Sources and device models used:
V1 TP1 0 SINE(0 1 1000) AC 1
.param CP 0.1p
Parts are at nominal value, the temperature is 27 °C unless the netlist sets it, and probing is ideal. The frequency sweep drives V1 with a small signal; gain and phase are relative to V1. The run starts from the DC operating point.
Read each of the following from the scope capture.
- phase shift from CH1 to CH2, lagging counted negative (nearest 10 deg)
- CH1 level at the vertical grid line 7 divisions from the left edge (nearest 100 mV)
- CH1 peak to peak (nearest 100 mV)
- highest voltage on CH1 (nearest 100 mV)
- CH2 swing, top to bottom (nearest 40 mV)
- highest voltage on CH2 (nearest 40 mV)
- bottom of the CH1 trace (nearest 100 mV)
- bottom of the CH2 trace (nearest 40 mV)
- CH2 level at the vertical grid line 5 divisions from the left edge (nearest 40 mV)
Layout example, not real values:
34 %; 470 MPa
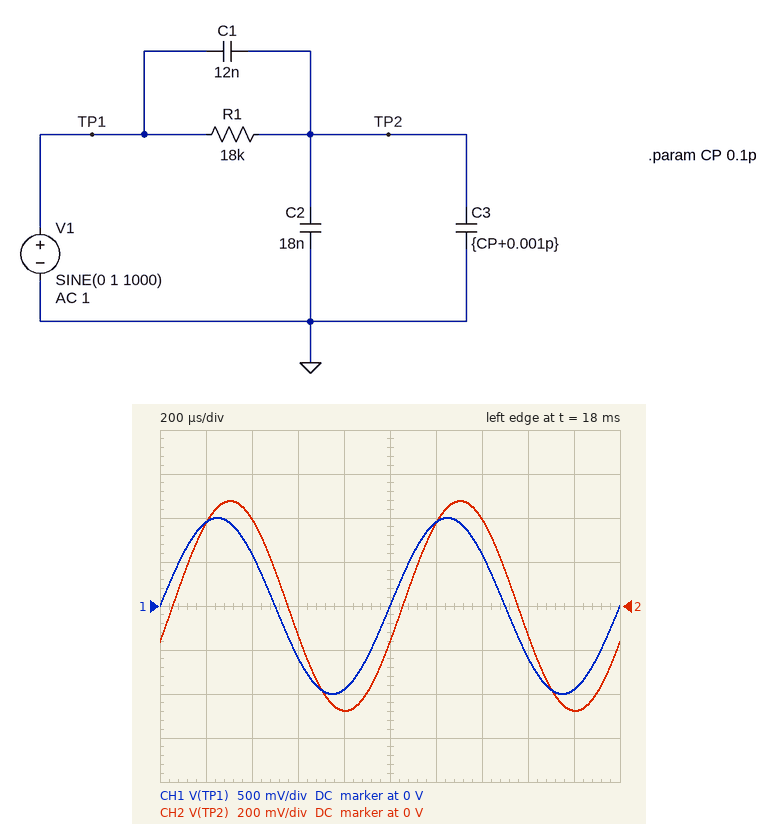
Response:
-20 deg; 600 mV; 2.0 V; 1.0 V; 960 mV; 480 mV; -1.0 V; -480 mV; -160 mV
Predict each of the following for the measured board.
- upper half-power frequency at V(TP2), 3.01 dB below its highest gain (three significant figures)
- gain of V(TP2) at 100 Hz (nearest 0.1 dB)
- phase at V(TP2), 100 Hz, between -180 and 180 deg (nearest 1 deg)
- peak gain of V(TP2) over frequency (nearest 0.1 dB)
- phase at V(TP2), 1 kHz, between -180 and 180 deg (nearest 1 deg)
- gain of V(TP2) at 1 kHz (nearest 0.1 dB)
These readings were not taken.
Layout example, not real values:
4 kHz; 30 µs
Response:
357 Hz; -0.4 dB; -11 deg; 0 dB; -20 deg; -6.4 dB
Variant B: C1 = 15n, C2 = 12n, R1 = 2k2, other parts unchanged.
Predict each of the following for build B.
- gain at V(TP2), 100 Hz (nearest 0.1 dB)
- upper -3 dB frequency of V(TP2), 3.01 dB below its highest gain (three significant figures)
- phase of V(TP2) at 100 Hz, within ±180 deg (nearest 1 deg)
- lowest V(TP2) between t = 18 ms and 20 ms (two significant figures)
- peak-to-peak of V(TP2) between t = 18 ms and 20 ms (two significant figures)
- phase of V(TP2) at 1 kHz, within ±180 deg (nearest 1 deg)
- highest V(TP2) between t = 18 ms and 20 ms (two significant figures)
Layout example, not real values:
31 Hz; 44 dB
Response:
0 dB; 4.33 kHz; -1 deg; -960 mV; 1.9 V; -9 deg; 960 mV
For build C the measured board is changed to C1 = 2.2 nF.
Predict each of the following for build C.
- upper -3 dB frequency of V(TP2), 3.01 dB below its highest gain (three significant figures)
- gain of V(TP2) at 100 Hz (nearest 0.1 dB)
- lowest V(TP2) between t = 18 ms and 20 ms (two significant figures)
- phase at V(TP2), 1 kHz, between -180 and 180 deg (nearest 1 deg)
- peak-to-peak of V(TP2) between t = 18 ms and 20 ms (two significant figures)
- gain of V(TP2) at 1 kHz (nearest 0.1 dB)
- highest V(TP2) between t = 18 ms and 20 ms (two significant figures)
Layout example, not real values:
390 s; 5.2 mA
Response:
443 Hz; -0.2 dB; -410 mV; -52 deg; 830 mV; -7.7 dB; 410 mV
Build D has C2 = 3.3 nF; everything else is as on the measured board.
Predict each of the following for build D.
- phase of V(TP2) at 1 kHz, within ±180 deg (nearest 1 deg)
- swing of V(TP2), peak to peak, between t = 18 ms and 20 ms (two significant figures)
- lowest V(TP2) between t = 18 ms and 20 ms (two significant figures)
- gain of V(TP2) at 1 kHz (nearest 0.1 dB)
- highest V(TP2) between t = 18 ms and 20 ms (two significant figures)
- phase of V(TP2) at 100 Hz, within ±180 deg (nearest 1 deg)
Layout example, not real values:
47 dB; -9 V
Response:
-6 deg; 1.7 V; -840 mV; -1.5 dB; 840 mV; -2 deg
